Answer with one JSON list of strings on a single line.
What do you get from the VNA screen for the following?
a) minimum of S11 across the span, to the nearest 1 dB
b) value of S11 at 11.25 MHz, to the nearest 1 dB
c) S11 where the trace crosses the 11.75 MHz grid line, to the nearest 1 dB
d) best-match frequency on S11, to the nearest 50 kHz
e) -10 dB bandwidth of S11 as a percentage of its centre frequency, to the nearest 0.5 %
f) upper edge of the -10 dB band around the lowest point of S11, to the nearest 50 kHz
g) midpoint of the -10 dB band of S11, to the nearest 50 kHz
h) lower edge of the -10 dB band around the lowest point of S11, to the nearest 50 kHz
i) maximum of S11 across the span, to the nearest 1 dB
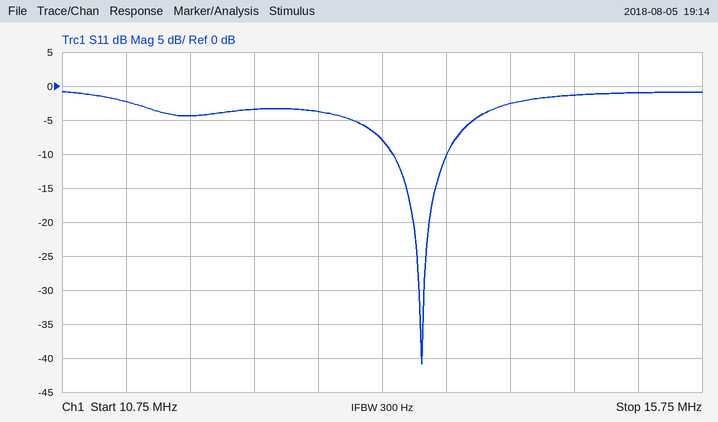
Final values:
["-41 dB", "-2 dB", "-4 dB", "13.55 MHz", "3.0 %", "13.75 MHz", "13.55 MHz", "13.35 MHz", "-1 dB"]
